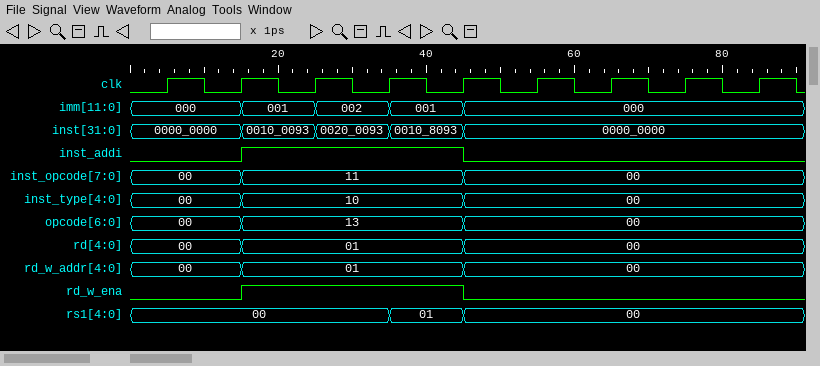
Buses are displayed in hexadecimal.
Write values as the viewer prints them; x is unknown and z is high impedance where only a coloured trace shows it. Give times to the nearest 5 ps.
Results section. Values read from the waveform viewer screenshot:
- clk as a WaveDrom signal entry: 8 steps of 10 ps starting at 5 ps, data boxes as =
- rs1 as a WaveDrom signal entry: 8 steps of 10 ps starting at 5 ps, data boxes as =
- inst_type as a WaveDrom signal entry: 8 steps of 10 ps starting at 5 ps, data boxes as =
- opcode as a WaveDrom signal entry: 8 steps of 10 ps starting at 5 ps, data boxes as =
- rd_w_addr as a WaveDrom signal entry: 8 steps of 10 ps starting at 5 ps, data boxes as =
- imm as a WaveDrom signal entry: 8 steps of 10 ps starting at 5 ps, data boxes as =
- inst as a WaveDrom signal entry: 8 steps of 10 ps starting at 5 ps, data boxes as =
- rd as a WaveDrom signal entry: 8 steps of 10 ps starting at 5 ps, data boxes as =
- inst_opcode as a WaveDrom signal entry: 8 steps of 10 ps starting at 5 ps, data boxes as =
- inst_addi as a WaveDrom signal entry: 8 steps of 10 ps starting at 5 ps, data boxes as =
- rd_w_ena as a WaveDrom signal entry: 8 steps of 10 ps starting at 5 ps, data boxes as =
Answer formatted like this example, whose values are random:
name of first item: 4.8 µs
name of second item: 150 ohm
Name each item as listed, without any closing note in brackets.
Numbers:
clk as a WaveDrom signal entry: 8 steps of 10 ps starting at 5 ps, data boxes as =: {name: 'clk', wave: 'p.......'}
rs1 as a WaveDrom signal entry: 8 steps of 10 ps starting at 5 ps, data boxes as =: {name: 'rs1', wave: '=..==...', data: '00 01 00'}
inst_type as a WaveDrom signal entry: 8 steps of 10 ps starting at 5 ps, data boxes as =: {name: 'inst_type', wave: '==..=...', data: '00 10 00'}
opcode as a WaveDrom signal entry: 8 steps of 10 ps starting at 5 ps, data boxes as =: {name: 'opcode', wave: '==..=...', data: '00 13 00'}
rd_w_addr as a WaveDrom signal entry: 8 steps of 10 ps starting at 5 ps, data boxes as =: {name: 'rd_w_addr', wave: '==..=...', data: '00 01 00'}
imm as a WaveDrom signal entry: 8 steps of 10 ps starting at 5 ps, data boxes as =: {name: 'imm', wave: '=====...', data: '000 001 002 001 000'}
inst as a WaveDrom signal entry: 8 steps of 10 ps starting at 5 ps, data boxes as =: {name: 'inst', wave: '=====...', data: '0000_0000 0010_0093 0020_0093 0010_8093 0000_0000'}
rd as a WaveDrom signal entry: 8 steps of 10 ps starting at 5 ps, data boxes as =: {name: 'rd', wave: '==..=...', data: '00 01 00'}
inst_opcode as a WaveDrom signal entry: 8 steps of 10 ps starting at 5 ps, data boxes as =: {name: 'inst_opcode', wave: '==..=...', data: '00 11 00'}
inst_addi as a WaveDrom signal entry: 8 steps of 10 ps starting at 5 ps, data boxes as =: {name: 'inst_addi', wave: '01..0...'}
rd_w_ena as a WaveDrom signal entry: 8 steps of 10 ps starting at 5 ps, data boxes as =: {name: 'rd_w_ena', wave: '01..0...'}
